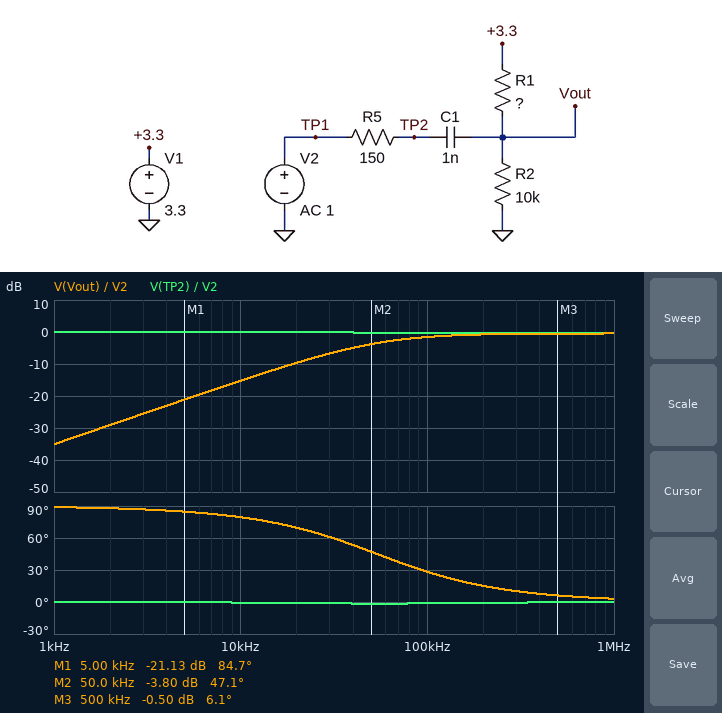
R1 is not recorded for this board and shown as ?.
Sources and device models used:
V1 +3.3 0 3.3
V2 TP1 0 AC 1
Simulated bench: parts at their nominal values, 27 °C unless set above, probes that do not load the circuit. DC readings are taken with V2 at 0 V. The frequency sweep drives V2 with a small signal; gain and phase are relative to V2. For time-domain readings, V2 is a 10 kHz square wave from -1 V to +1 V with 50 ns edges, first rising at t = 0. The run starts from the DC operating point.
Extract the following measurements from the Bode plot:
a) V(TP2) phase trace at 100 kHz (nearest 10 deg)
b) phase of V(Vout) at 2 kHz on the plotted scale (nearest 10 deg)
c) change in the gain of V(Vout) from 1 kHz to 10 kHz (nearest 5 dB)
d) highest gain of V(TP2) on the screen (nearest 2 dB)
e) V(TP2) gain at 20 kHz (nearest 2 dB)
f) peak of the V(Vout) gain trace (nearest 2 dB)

0 deg
90 deg
20 dB
0 dB
0 dB
0 dB
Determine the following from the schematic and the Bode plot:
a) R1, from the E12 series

3.9 kΩ
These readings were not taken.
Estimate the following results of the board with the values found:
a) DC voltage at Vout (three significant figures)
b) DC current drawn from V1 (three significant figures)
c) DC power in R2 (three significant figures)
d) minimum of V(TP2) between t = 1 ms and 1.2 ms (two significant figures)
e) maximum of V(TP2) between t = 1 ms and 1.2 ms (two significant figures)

2.37 V
237 µA
564 µW
-1.0 V
1.0 V
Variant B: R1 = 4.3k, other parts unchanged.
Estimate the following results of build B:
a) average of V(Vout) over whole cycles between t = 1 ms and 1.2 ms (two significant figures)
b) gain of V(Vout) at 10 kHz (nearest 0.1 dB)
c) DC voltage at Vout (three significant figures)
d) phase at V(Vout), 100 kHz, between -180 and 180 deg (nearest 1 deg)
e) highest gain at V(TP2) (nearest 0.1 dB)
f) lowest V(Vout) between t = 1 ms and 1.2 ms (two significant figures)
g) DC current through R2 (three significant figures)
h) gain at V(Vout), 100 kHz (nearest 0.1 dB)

2.3 V
-14.6 dB
2.31 V
27 deg
0 dB
420 mV
231 µA
-1.4 dB
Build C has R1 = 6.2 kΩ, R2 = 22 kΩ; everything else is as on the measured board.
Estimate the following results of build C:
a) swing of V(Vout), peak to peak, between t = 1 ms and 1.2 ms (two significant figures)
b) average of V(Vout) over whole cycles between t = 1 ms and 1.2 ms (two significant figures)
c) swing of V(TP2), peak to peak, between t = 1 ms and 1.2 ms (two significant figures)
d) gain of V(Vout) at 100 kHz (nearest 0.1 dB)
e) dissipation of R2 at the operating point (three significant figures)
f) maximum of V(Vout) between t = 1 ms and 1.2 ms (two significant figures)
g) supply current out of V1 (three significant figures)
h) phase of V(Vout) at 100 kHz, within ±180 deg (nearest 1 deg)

3.9 V
2.6 V
2.0 V
-0.7 dB
301 µW
4.5 V
117 µA
18 deg
